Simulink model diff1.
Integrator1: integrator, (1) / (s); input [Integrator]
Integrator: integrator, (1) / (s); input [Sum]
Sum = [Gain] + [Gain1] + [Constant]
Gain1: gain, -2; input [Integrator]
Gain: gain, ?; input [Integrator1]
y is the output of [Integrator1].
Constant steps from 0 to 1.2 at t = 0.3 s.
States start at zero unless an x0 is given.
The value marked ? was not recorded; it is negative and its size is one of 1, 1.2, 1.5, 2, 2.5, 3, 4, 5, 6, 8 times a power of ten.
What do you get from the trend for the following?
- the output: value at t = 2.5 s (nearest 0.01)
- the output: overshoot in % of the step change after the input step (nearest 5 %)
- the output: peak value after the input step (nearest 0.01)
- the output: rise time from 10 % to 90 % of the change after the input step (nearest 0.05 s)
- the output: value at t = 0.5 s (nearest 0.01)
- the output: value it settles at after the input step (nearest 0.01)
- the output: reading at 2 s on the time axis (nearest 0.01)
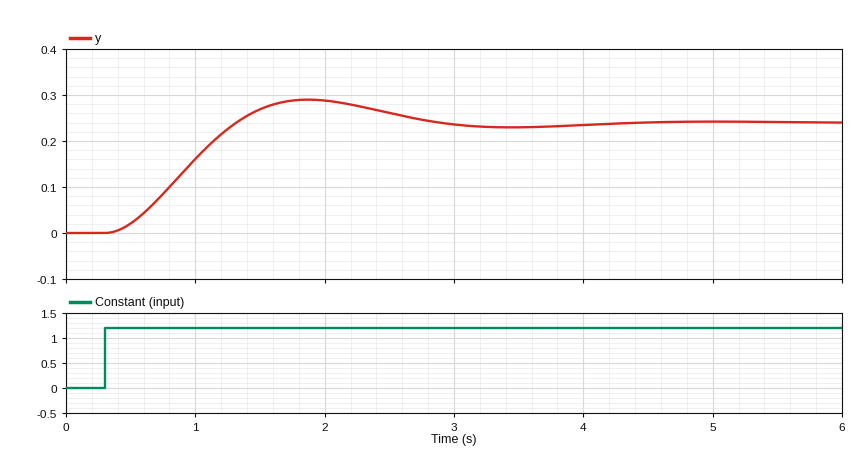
0.26
20 %
0.29
0.70 s
0.02
0.24
0.29
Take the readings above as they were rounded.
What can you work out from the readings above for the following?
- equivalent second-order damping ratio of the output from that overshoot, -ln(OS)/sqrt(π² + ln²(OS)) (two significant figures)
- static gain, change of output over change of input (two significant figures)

0.46
0.20
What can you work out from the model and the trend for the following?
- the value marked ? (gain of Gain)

-5
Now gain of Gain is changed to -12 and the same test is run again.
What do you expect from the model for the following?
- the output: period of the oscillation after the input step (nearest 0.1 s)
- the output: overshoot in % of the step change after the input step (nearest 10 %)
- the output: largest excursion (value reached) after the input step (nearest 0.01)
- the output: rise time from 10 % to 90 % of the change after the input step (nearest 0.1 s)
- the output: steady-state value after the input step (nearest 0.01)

1.9 s
40 %
0.14
0.4 s
0.10
